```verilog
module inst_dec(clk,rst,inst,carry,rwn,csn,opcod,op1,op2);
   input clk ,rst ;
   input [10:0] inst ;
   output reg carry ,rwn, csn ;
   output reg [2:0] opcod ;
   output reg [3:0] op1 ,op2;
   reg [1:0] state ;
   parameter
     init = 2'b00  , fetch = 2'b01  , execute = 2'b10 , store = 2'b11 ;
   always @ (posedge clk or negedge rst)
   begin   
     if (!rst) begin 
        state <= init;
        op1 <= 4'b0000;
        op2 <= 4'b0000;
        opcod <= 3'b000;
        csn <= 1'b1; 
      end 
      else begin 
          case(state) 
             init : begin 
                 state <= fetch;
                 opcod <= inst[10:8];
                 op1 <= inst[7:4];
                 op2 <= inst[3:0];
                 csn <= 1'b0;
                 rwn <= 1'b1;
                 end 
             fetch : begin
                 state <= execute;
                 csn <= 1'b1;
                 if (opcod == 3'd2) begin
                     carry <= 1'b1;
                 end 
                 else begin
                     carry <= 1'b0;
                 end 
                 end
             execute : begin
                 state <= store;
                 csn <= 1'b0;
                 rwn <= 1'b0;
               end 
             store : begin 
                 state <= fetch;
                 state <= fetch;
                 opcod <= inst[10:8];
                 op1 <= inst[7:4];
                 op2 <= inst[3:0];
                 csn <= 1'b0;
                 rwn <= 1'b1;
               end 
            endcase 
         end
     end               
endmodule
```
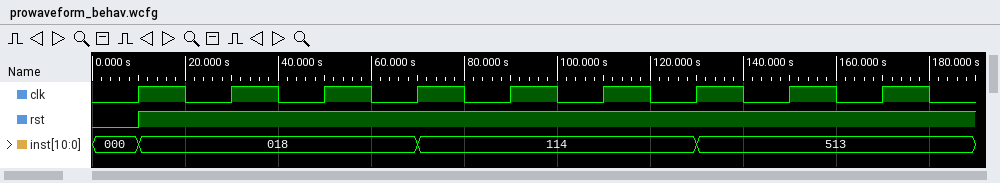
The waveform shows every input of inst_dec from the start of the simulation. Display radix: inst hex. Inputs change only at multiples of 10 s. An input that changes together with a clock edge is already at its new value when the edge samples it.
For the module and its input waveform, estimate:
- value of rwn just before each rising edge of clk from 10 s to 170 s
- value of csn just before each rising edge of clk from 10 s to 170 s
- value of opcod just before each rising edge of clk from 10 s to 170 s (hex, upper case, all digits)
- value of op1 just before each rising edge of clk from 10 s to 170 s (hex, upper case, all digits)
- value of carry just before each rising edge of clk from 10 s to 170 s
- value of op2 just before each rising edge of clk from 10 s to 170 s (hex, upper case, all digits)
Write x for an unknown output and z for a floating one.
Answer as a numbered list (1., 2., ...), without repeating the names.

1. x 1 1 0 1 1 0 1 1
2. 1 0 1 0 0 1 0 0 1
3. 0, 0, 0, 0, 1, 1, 1, 5, 5
4. 0, 1, 1, 1, 1, 1, 1, 1, 1
5. x x 0 0 0 0 0 0 0
6. 0, 8, 8, 8, 4, 4, 4, 3, 3
